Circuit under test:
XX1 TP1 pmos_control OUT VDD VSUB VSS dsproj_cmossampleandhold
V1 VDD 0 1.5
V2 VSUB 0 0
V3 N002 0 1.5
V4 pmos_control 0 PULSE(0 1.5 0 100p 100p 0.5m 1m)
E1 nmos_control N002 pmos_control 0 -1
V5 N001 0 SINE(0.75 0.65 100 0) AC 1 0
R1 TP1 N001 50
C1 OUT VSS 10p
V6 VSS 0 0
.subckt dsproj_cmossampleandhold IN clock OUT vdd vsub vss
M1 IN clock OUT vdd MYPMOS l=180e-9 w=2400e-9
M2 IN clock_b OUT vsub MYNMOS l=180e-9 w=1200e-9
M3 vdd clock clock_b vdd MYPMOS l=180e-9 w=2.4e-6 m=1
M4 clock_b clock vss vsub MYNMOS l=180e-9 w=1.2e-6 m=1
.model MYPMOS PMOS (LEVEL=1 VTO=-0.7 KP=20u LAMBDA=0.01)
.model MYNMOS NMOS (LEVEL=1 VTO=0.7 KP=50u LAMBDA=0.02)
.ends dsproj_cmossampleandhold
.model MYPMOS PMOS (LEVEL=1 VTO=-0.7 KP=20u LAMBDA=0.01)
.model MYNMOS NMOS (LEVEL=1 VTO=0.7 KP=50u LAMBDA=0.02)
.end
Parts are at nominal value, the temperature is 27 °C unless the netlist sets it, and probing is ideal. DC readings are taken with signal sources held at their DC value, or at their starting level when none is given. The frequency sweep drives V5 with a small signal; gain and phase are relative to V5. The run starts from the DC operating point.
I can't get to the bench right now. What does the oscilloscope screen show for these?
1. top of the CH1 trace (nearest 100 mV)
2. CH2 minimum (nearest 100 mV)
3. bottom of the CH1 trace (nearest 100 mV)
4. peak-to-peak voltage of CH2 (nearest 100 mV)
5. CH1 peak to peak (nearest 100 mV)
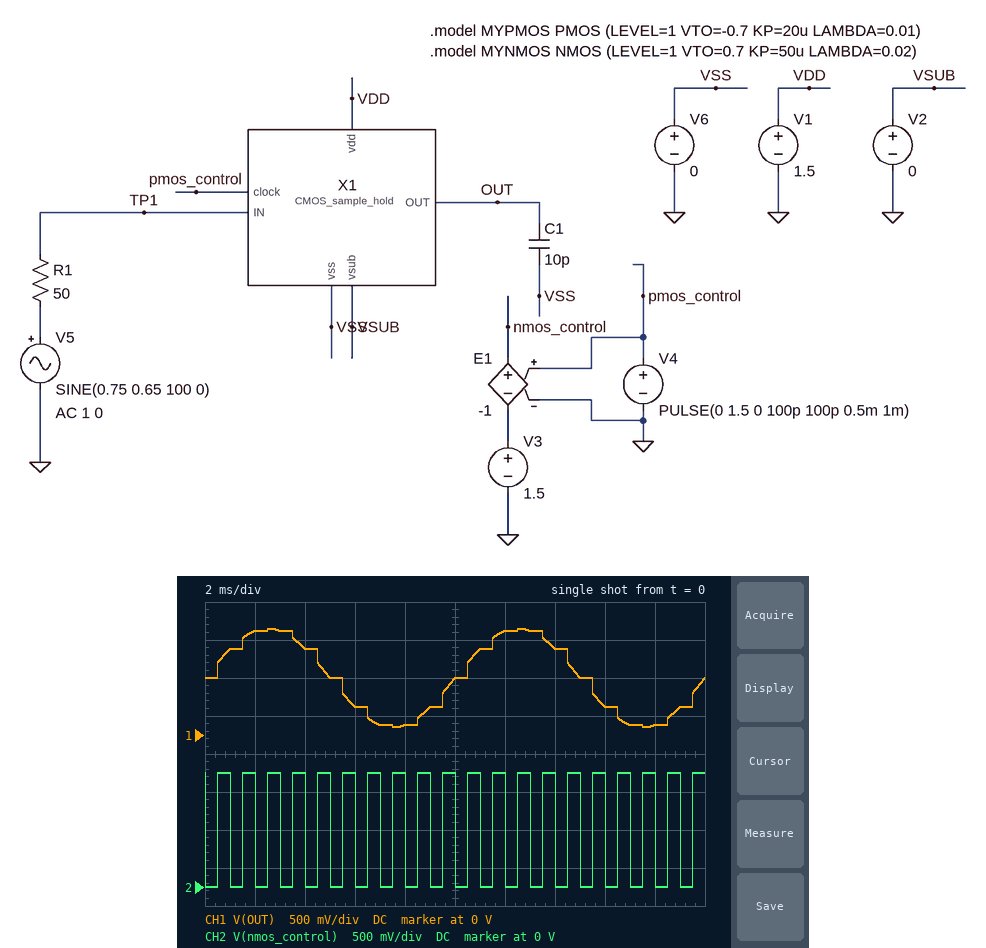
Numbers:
1.4 V
0 V
100 mV
1.5 V
1.3 V
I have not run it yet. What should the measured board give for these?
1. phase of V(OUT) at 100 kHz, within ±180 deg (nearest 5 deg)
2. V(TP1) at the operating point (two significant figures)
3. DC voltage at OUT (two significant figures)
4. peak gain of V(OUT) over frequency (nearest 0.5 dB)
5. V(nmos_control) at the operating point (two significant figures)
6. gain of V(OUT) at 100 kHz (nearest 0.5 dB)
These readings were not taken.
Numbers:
-10 deg
750 mV
750 mV
0 dB
1.5 V
0 dB
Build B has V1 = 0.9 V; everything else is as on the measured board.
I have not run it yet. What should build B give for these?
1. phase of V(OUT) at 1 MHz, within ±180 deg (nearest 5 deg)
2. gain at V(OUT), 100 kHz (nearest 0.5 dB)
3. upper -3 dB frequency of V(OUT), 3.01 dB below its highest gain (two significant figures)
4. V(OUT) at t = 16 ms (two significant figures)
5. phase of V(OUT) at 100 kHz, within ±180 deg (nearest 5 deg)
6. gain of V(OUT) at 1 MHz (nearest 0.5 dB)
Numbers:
-80 deg
-1.0 dB
210 kHz
700 mV
-25 deg
-13.5 dB
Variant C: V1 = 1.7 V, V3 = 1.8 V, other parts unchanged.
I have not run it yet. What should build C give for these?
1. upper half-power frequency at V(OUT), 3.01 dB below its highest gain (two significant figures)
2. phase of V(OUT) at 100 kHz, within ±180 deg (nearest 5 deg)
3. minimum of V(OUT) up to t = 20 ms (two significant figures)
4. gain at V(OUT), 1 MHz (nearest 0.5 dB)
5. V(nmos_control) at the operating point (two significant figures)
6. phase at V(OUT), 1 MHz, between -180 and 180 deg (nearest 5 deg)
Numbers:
1.5 MHz
-5 deg
100 mV
-1.5 dB
1.8 V
-35 deg
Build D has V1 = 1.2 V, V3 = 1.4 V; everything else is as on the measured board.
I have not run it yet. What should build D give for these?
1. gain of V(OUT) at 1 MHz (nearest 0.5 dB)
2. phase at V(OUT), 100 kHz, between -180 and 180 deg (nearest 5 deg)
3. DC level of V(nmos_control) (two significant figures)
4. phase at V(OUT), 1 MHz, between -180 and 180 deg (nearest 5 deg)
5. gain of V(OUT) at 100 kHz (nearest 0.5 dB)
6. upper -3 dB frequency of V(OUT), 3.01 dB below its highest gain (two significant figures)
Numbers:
-13.5 dB
-25 deg
1.4 V
-80 deg
-1.0 dB
210 kHz
